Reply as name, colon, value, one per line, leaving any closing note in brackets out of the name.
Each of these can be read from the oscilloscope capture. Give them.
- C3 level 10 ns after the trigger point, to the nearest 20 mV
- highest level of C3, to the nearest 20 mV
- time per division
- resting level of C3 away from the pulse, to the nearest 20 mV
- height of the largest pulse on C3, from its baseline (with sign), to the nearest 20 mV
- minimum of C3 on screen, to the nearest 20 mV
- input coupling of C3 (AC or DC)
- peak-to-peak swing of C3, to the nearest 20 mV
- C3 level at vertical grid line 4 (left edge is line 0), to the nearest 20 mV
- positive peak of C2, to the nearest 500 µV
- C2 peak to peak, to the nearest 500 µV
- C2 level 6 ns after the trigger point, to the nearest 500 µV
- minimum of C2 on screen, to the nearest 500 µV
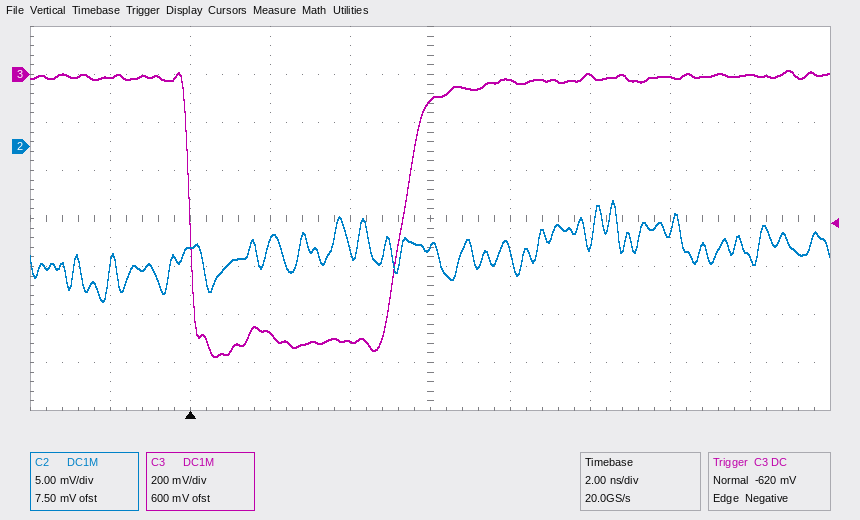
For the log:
C3 level 10 ns after the trigger point, to the nearest 20 mV: 0 mV
highest level of C3, to the nearest 20 mV: 20 mV
time per division: 2 ns
resting level of C3 away from the pulse, to the nearest 20 mV: -20 mV
height of the largest pulse on C3, from its baseline (with sign), to the nearest 20 mV: -1.16 V
minimum of C3 on screen, to the nearest 20 mV: -1.18 V
input coupling of C3: DC
peak-to-peak swing of C3, to the nearest 20 mV: 1.20 V
C3 level at vertical grid line 4 (left edge is line 0), to the nearest 20 mV: -1.12 V
positive peak of C2, to the nearest 500 µV: -5.5 mV
C2 peak to peak, to the nearest 500 µV: 10.5 mV
C2 level 6 ns after the trigger point, to the nearest 500 µV: -10.5 mV
minimum of C2 on screen, to the nearest 500 µV: -16.0 mV
